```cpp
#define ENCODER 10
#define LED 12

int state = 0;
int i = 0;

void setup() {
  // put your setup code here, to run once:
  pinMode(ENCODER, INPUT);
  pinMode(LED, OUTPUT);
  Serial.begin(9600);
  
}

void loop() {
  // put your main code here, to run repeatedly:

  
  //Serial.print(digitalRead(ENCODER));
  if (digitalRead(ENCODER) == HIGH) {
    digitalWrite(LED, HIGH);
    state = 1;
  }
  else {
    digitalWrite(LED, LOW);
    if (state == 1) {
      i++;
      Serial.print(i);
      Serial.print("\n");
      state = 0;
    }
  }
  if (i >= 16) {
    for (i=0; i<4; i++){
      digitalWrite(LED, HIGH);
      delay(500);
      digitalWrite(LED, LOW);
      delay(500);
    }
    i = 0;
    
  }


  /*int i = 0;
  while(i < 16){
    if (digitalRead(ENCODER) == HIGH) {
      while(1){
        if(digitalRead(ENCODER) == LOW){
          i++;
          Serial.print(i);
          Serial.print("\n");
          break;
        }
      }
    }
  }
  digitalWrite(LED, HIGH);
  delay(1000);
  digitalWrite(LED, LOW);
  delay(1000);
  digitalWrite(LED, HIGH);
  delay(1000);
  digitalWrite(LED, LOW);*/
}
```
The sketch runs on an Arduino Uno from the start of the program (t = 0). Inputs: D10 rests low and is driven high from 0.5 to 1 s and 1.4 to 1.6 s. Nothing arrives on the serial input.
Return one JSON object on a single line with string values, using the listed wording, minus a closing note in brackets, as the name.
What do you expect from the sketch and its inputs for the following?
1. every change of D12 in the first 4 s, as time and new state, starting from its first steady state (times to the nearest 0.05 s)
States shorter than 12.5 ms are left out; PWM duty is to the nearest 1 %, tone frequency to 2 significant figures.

{"every change of D12 in the first 4 s, as time and new state, starting from its first steady state": "0 s low; 0.5 s high; 1 s low; 1.4 s high; 1.6 s low"}
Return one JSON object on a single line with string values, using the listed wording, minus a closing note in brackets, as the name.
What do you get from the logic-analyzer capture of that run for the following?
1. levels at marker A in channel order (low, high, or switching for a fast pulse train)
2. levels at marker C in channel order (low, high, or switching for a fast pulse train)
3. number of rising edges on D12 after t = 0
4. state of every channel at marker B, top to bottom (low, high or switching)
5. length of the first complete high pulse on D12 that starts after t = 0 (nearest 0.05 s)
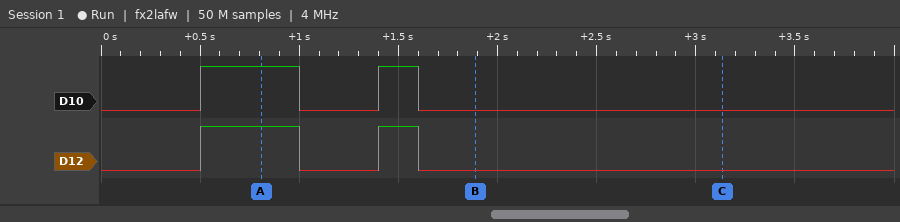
{"levels at marker A in channel order": "D10 high, D12 high", "levels at marker C in channel order": "D10 low, D12 low", "number of rising edges on D12 after t = 0": "2", "state of every channel at marker B, top to bottom": "D10 low, D12 low", "length of the first complete high pulse on D12 that starts after t = 0": "0.50 s"}
